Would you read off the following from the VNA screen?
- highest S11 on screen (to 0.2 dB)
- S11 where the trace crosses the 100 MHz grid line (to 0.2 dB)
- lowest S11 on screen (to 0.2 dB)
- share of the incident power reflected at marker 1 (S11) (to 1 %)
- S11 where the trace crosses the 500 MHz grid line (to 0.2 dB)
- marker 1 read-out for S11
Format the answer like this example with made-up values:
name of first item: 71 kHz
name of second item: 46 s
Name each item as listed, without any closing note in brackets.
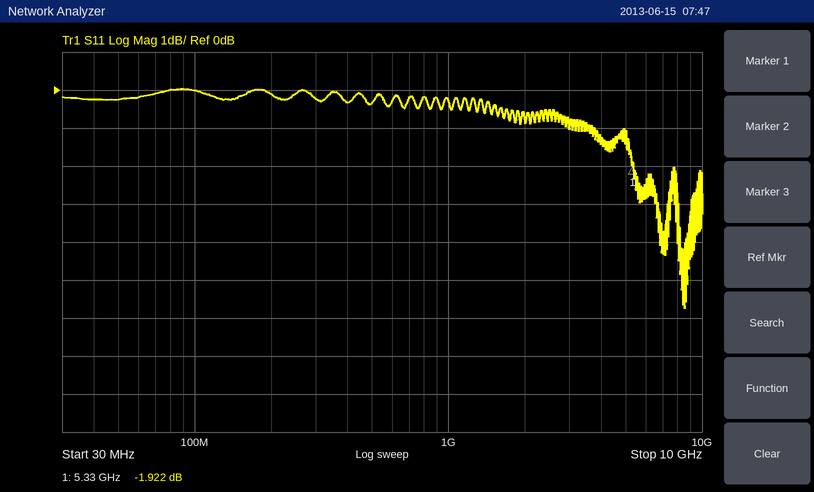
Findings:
highest S11 on screen: 0.0 dB
S11 where the trace crosses the 100 MHz grid line: 0.0 dB
lowest S11 on screen: -5.8 dB
share of the incident power reflected at marker 1 (S11): 64 %
S11 where the trace crosses the 500 MHz grid line: -0.4 dB
marker 1 read-out for S11: -1.922 dB
